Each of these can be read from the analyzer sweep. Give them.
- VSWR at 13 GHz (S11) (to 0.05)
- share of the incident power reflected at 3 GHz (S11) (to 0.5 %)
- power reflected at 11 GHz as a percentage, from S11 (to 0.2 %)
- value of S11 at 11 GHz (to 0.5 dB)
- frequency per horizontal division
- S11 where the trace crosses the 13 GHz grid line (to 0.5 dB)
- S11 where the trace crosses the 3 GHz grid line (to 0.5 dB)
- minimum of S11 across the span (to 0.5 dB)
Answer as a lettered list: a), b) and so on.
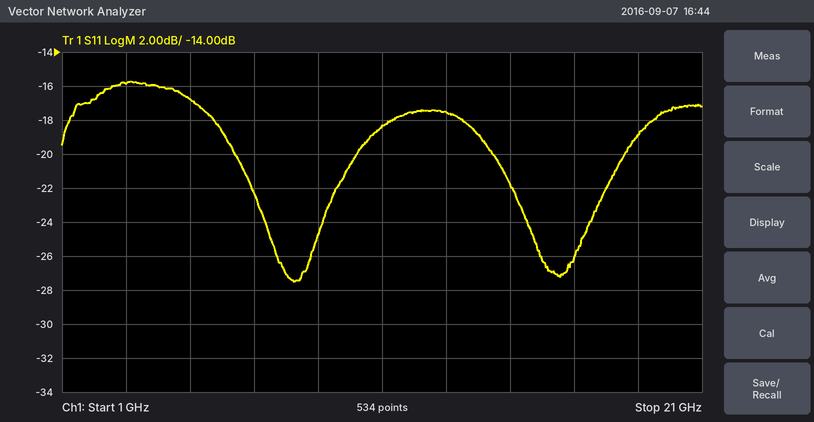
a) 1.30
b) 2.5 %
c) 1.4 %
d) -18.5 dB
e) 2 GHz
f) -17.5 dB
g) -16.0 dB
h) -27.5 dB
